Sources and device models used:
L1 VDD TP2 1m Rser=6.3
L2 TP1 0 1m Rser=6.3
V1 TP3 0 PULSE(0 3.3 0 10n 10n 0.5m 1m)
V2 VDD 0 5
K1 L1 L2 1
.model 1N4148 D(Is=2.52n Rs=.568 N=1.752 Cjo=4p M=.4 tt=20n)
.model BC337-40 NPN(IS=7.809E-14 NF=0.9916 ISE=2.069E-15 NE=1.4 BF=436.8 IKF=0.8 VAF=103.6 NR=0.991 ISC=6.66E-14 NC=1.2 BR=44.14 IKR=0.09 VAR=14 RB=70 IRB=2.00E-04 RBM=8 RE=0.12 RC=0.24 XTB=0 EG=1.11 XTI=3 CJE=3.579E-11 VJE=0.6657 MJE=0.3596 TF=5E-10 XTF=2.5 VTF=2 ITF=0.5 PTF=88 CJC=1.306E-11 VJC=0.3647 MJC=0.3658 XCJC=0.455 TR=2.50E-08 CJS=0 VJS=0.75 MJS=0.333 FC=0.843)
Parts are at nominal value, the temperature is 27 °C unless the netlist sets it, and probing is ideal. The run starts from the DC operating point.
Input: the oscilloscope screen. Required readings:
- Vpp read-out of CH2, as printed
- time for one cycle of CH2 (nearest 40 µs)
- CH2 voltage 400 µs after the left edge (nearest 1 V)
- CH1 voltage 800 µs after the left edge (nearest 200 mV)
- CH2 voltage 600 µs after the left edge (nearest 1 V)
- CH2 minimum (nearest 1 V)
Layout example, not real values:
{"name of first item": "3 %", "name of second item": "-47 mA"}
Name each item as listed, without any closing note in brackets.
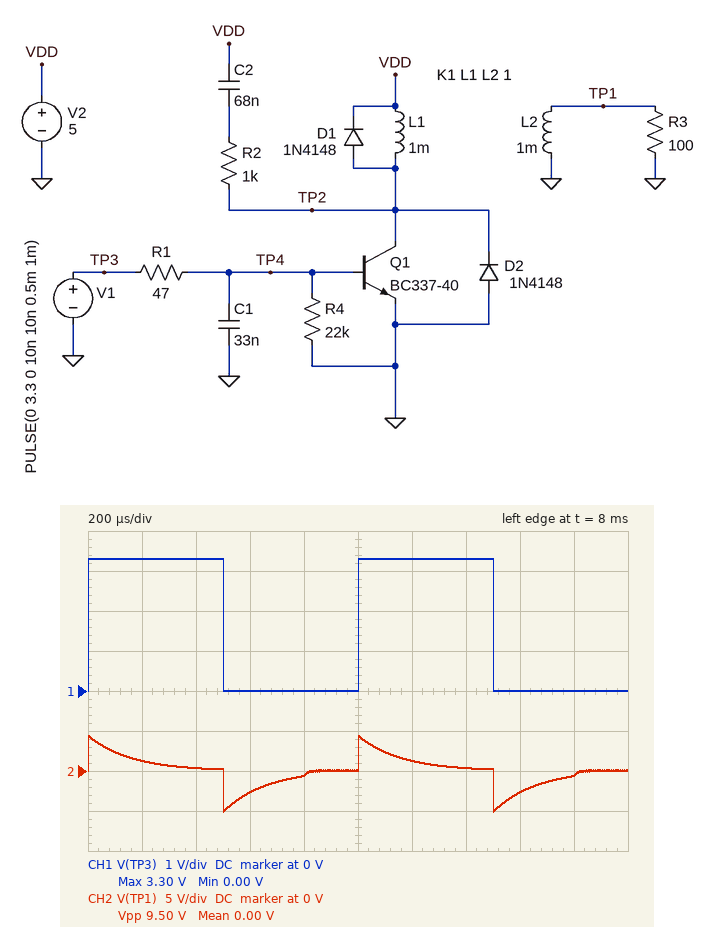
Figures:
{"Vpp read-out of CH2, as printed": "9.50 V", "time for one cycle of CH2": "1.00 ms", "CH2 voltage 400 µs after the left edge": "0 V", "CH1 voltage 800 µs after the left edge": "0 V", "CH2 voltage 600 µs after the left edge": "-3 V", "CH2 minimum": "-5 V"}
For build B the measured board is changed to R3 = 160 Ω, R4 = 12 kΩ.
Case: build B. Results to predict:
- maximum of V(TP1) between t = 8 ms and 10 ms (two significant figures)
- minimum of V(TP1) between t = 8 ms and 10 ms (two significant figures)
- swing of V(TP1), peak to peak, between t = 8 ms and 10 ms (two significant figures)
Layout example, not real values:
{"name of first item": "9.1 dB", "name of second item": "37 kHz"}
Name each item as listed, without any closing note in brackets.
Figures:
{"maximum of V(TP1) between t = 8 ms and 10 ms": "4.6 V", "minimum of V(TP1) between t = 8 ms and 10 ms": "-5.3 V", "swing of V(TP1), peak to peak, between t = 8 ms and 10 ms": "9.9 V"}
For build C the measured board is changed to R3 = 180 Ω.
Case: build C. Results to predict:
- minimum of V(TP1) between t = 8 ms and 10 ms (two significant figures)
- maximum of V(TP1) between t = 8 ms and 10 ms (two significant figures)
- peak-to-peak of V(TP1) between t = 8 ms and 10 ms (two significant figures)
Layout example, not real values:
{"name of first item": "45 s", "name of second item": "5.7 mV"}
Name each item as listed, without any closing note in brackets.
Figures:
{"minimum of V(TP1) between t = 8 ms and 10 ms": "-5.4 V", "maximum of V(TP1) between t = 8 ms and 10 ms": "4.6 V", "peak-to-peak of V(TP1) between t = 8 ms and 10 ms": "10 V"}
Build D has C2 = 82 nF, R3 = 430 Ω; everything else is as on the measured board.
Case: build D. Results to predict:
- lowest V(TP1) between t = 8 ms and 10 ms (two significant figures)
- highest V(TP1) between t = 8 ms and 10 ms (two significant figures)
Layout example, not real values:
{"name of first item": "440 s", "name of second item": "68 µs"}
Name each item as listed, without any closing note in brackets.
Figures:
{"lowest V(TP1) between t = 8 ms and 10 ms": "-5.6 V", "highest V(TP1) between t = 8 ms and 10 ms": "4.8 V"}
